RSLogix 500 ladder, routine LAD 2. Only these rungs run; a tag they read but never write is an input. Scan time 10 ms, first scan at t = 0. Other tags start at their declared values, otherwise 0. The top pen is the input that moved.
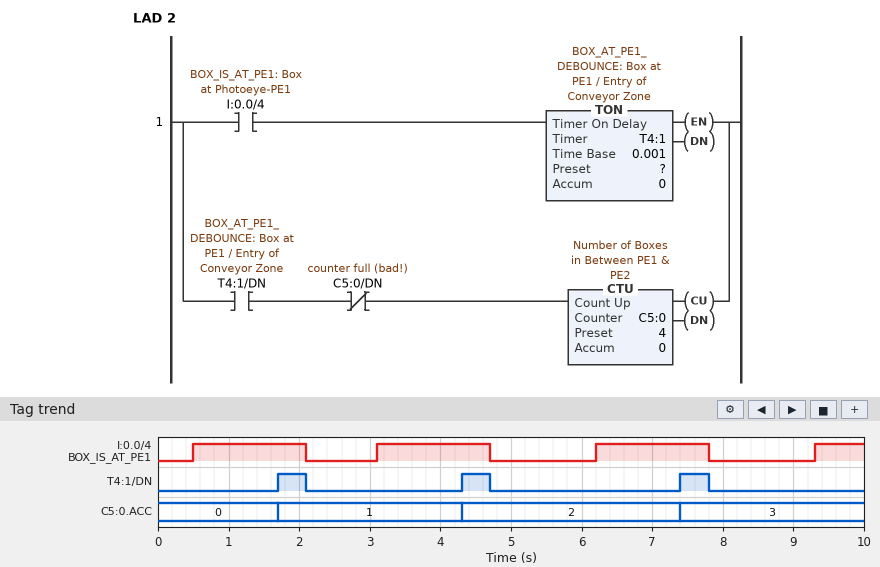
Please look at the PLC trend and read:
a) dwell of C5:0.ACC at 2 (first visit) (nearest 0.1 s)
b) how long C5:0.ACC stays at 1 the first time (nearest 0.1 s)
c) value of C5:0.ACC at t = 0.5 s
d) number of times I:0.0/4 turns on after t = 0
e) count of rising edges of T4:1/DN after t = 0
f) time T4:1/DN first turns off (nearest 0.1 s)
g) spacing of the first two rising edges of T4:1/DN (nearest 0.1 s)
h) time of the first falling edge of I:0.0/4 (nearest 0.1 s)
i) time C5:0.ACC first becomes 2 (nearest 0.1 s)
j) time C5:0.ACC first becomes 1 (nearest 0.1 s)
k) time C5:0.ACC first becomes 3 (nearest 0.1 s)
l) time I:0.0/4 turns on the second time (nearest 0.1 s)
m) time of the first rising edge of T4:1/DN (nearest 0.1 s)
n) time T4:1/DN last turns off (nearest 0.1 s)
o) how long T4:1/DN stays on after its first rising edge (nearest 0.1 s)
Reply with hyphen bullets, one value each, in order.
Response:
- 3.1 s
- 2.6 s
- 0
- 4
- 3
- 2.1 s
- 2.6 s
- 2.1 s
- 4.3 s
- 1.7 s
- 7.4 s
- 3.1 s
- 1.7 s
- 7.8 s
- 0.4 s
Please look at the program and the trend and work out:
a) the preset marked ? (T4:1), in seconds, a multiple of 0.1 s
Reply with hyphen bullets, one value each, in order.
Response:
- 1.2 s
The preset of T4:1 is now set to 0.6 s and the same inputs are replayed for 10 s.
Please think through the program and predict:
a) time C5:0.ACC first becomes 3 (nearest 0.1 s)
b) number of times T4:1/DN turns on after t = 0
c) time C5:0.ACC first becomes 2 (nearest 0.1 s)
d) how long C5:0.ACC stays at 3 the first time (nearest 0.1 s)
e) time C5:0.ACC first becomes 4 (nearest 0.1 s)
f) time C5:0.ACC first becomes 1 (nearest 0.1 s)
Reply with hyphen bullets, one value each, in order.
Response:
- 6.8 s
- 4
- 3.7 s
- 3.1 s
- 9.9 s
- 1.1 s
